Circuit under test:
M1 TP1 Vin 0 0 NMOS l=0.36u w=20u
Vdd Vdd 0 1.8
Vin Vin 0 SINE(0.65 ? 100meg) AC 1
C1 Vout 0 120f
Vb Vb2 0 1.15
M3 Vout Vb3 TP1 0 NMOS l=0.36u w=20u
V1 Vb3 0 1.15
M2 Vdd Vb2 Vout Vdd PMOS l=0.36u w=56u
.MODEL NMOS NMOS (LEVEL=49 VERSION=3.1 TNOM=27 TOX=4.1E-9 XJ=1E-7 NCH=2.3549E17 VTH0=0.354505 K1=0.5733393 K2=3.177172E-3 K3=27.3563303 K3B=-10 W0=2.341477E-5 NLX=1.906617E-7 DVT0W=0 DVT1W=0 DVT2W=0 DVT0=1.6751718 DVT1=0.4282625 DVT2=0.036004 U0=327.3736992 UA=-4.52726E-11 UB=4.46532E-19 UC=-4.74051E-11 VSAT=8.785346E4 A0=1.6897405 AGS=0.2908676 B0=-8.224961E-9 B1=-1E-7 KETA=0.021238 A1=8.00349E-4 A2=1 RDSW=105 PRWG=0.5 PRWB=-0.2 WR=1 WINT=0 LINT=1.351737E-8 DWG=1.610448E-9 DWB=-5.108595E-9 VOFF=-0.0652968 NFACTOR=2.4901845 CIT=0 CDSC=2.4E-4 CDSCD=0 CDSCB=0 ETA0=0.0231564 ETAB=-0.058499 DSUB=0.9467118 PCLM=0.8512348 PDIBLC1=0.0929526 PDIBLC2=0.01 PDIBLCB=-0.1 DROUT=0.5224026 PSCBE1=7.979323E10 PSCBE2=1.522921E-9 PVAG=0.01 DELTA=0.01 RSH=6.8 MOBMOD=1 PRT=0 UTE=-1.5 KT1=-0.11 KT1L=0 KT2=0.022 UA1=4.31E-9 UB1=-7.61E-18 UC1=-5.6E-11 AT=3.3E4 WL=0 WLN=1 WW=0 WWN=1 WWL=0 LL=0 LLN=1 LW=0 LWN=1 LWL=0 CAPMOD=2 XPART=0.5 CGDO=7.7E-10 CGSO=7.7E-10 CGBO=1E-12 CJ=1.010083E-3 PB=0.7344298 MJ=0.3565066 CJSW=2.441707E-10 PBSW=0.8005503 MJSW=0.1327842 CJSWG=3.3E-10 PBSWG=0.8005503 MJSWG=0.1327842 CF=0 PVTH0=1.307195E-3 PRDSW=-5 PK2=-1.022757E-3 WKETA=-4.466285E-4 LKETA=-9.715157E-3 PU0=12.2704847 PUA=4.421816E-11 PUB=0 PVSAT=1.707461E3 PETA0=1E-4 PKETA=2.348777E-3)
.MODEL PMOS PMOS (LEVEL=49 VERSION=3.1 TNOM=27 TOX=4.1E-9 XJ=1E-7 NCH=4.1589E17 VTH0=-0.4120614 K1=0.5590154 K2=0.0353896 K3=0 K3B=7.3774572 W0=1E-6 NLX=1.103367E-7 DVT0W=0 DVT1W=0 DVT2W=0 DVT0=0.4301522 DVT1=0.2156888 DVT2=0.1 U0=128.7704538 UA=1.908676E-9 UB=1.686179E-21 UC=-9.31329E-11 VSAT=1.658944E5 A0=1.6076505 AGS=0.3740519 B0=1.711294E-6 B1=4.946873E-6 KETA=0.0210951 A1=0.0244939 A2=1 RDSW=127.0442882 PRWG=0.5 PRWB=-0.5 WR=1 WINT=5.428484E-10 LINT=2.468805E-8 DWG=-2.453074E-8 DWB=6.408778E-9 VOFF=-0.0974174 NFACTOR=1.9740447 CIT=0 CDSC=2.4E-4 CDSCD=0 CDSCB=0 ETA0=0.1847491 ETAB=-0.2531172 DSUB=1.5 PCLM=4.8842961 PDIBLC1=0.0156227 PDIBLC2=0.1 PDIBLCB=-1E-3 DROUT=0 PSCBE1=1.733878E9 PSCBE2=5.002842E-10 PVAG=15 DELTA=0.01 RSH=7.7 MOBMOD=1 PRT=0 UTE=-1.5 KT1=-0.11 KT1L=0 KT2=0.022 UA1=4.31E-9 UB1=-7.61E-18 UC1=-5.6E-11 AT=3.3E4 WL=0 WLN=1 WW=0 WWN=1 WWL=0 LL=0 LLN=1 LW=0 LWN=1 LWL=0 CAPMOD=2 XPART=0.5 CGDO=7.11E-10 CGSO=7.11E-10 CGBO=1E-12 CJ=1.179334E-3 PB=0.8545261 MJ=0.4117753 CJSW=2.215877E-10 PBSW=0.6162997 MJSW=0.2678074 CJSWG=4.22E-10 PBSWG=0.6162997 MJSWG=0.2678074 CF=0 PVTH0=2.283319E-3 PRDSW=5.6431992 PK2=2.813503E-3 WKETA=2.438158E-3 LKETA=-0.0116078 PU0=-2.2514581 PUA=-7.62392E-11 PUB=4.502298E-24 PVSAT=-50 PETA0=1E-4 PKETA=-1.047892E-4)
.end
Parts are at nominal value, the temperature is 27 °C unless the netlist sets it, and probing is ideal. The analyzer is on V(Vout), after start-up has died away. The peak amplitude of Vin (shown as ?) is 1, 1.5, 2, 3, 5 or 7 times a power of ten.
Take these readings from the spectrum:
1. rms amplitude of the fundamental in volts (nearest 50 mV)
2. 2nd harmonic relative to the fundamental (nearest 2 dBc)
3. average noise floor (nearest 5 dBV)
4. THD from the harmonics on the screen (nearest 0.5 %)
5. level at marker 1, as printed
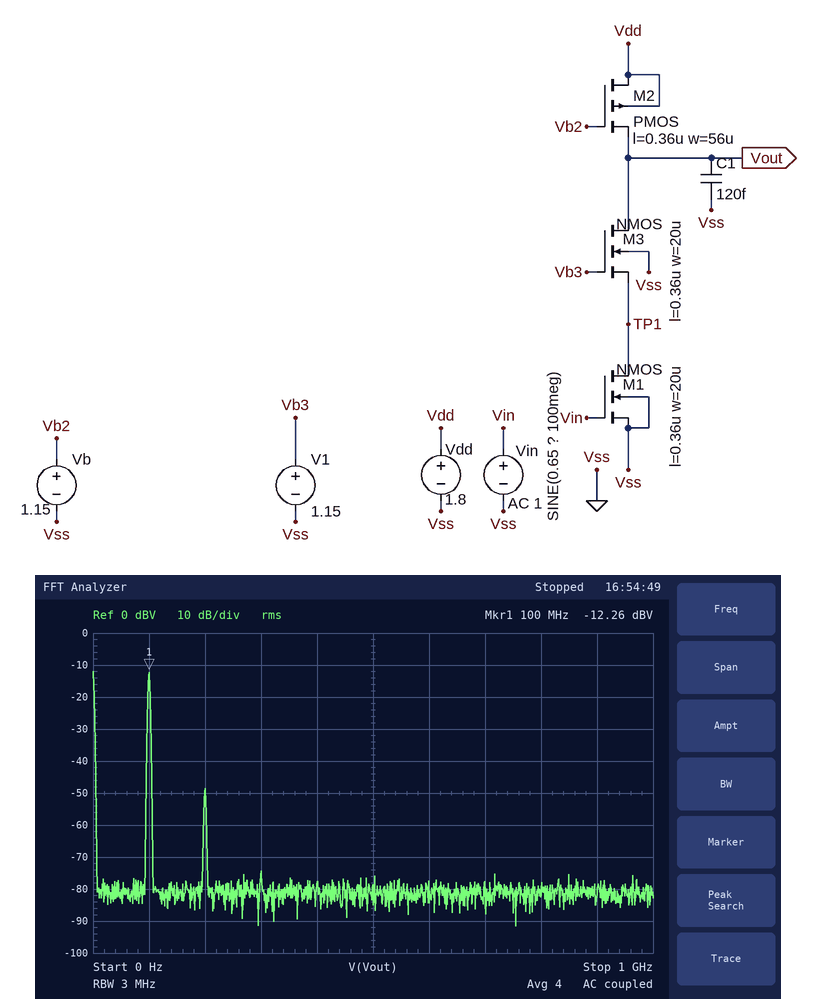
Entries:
250 mV
-36 dBc
-80 dBV
1.5 %
-12.26 dBV
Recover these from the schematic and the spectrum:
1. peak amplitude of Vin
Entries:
20 mV
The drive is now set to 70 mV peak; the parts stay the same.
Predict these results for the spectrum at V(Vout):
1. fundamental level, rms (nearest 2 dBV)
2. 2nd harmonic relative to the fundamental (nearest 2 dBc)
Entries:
-4 dBV
-18 dBc
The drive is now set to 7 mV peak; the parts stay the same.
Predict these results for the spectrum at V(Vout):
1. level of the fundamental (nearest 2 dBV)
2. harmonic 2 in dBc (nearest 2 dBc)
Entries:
-22 dBV
-46 dBc
